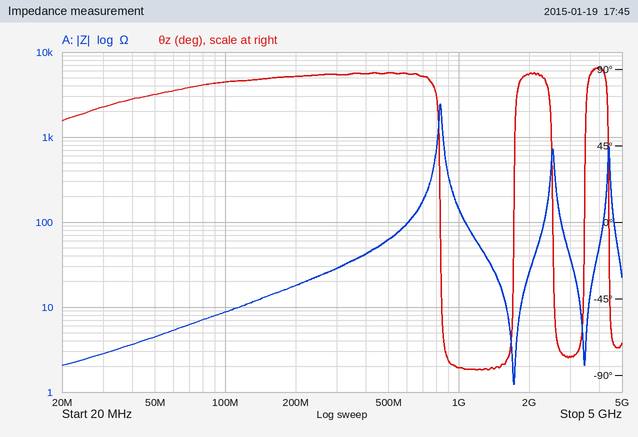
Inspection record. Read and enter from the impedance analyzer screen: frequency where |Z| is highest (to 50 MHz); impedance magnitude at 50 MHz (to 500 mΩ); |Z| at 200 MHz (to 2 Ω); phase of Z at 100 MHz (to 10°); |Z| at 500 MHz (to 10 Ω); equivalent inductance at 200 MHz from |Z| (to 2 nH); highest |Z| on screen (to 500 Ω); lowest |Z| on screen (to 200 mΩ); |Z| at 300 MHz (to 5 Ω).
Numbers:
850 MHz
4.5 Ω
18 Ω
80°
60 Ω
14 nH
2.5 kΩ
1.2 Ω
30 Ω
